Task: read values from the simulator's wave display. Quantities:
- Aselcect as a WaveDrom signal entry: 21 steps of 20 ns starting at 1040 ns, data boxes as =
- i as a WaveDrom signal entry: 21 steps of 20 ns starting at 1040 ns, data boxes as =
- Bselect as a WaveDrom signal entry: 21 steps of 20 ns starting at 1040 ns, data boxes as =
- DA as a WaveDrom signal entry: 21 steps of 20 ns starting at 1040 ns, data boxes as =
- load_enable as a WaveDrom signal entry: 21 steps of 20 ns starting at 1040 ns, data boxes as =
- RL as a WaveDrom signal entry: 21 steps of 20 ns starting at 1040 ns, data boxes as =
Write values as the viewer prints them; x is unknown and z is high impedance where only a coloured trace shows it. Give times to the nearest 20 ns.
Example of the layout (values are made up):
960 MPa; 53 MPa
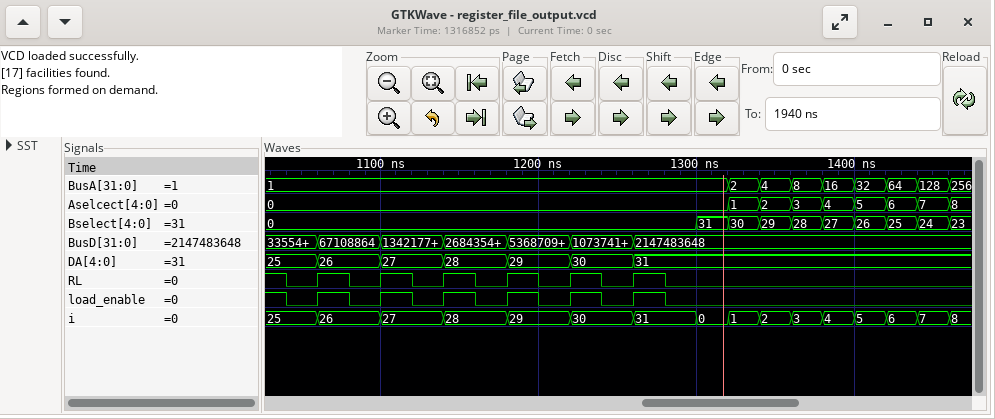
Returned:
{name: 'Aselcect', wave: '=.............=======', data: '0 1 2 3 4 5 6 7'}; {name: 'i', wave: '==.=.=.=.=.=.========', data: '25 26 27 28 29 30 31 0 1 2 3 4 5 6 7'}; {name: 'Bselect', wave: '=............========', data: '0 31 30 29 28 27 26 25 24'}; {name: 'DA', wave: '==.=.=.=.=.=.........', data: '25 26 27 28 29 30 31'}; {name: 'load_enable', wave: '0101010101010........'}; {name: 'RL', wave: '0101010101010........'}
